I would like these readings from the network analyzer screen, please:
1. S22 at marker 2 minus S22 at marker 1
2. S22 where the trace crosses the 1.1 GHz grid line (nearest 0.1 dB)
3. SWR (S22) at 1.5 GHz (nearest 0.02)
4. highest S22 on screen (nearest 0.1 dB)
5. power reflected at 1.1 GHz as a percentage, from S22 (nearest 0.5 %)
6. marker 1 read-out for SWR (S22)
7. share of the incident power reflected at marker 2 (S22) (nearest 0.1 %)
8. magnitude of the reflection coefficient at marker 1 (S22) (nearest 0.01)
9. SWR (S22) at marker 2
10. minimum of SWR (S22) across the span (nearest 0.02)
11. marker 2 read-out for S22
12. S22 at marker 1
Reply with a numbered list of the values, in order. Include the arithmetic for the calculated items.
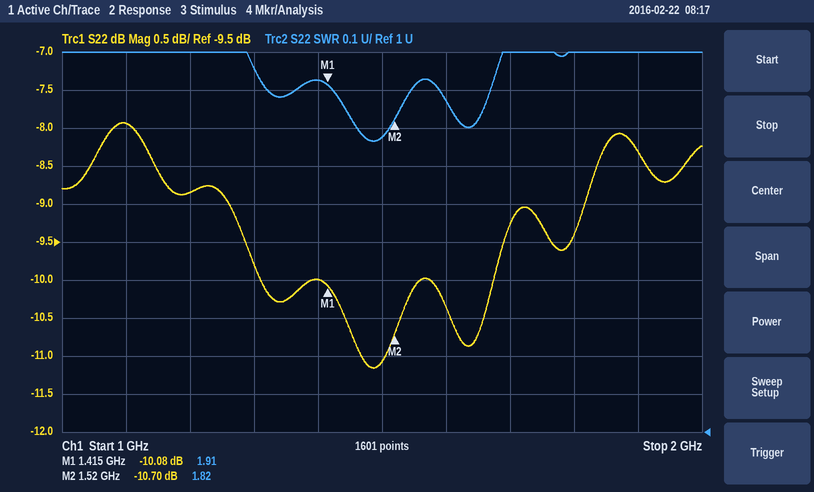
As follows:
1. -10.7 − (-10.08) = -0.62 dB
2. -7.9 dB
3. 1.78
4. -7.9 dB
5. 10^(-7.9/10) ≈ 16.2 %, so 16.0 % to the nearest 0.5 %
6. 1.91
7. 10^(-10.7/10) ≈ 8.5 %
8. 10^(-10.08/20) ≈ 0.31
9. 1.82
10. 1.76
11. -10.70 dB
12. -10.08 dB
